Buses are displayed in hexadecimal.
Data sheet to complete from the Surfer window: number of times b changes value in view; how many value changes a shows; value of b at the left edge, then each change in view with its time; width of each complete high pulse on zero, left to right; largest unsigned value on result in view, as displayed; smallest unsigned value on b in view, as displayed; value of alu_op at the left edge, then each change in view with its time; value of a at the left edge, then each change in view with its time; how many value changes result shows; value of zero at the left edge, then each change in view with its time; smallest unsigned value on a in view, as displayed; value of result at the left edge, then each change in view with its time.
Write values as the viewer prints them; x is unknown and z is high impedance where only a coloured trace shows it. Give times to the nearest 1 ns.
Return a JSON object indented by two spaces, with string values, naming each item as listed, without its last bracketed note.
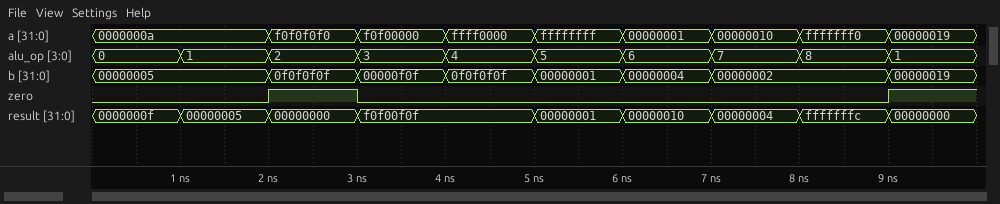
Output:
{
  "number of times b changes value in view": "7",
  "how many value changes a shows": "8",
  "value of b at the left edge, then each change in view with its time": "00000005, 0f0f0f0f at 2 ns, 00000f0f at 3 ns, 0f0f0f0f at 4 ns, 00000001 at 5 ns, 00000004 at 6 ns, 00000002 at 7 ns, 00000019 at 9 ns",
  "width of each complete high pulse on zero, left to right": "1 ns",
  "largest unsigned value on result in view, as displayed": "fffffffc",
  "smallest unsigned value on b in view, as displayed": "00000001",
  "value of alu_op at the left edge, then each change in view with its time": "0, 1 at 1 ns, 2 at 2 ns, 3 at 3 ns, 4 at 4 ns, 5 at 5 ns, 6 at 6 ns, 7 at 7 ns, 8 at 8 ns, 1 at 9 ns",
  "value of a at the left edge, then each change in view with its time": "0000000a, f0f0f0f0 at 2 ns, f0f00000 at 3 ns, ffff0000 at 4 ns, ffffffff at 5 ns, 00000001 at 6 ns, 00000010 at 7 ns, fffffff0 at 8 ns, 00000019 at 9 ns",
  "how many value changes result shows": "8",
  "value of zero at the left edge, then each change in view with its time": "0, 1 at 2 ns, 0 at 3 ns, 1 at 9 ns",
  "smallest unsigned value on a in view, as displayed": "00000001",
  "value of result at the left edge, then each change in view with its time": "0000000f, 00000005 at 1 ns, 00000000 at 2 ns, f0f00f0f at 3 ns, 00000001 at 5 ns, 00000010 at 6 ns, 00000004 at 7 ns, fffffffc at 8 ns, 00000000 at 9 ns"
}
